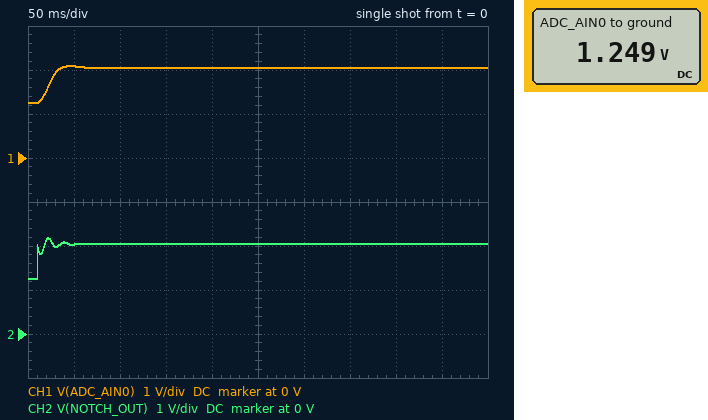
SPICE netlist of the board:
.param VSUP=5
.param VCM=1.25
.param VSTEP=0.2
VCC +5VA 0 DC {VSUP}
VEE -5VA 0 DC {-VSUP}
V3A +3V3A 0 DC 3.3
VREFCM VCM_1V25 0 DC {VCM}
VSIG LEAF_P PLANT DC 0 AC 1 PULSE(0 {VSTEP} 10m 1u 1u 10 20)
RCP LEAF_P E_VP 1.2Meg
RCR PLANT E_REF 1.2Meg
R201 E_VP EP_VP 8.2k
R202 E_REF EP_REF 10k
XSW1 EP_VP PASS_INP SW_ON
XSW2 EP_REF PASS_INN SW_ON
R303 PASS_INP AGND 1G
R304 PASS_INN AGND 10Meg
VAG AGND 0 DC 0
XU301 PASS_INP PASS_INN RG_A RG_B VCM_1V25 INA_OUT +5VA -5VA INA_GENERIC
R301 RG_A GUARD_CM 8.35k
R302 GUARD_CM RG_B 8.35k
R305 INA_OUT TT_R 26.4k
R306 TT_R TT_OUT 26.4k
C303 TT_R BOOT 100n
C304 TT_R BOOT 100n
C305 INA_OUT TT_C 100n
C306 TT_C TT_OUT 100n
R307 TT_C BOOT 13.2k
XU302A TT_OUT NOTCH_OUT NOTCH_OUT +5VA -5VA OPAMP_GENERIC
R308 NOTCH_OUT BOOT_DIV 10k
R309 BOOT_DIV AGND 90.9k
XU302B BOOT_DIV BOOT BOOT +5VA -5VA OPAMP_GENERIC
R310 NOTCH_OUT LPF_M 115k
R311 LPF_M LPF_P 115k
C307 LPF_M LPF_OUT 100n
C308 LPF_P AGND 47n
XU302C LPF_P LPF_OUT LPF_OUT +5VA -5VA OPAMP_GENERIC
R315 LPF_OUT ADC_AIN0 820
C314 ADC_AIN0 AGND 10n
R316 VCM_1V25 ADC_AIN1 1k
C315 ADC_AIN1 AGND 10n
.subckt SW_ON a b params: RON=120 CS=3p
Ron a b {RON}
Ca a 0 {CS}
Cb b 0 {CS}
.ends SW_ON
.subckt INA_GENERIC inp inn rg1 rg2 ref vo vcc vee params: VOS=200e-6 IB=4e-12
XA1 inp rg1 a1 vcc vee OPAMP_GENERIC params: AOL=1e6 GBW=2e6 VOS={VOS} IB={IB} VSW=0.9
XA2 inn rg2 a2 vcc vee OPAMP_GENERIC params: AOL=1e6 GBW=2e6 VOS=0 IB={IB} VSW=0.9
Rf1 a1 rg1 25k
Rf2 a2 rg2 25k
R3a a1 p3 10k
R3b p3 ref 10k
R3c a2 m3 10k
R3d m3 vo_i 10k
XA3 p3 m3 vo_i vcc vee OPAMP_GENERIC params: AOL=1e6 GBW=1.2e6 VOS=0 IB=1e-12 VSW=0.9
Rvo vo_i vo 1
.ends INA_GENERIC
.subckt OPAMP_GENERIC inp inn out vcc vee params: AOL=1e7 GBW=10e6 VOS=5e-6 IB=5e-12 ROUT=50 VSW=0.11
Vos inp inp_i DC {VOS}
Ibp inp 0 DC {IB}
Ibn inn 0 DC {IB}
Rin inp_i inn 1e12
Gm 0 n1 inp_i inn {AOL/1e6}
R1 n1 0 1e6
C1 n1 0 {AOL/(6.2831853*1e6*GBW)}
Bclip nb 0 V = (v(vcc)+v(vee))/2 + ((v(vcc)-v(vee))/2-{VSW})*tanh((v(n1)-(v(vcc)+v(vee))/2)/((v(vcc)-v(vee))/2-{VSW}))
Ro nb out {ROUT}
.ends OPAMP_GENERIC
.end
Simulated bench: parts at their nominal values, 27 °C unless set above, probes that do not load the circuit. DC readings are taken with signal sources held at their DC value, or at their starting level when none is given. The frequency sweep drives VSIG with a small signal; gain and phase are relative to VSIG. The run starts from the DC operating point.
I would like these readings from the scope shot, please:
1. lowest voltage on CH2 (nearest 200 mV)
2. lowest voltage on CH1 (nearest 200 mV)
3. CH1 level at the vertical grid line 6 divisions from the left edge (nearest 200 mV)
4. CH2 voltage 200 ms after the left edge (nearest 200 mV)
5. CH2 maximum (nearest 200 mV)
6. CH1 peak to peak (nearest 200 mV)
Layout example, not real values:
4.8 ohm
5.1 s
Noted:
1.2 V
1.2 V
2.0 V
2.0 V
2.2 V
800 mV
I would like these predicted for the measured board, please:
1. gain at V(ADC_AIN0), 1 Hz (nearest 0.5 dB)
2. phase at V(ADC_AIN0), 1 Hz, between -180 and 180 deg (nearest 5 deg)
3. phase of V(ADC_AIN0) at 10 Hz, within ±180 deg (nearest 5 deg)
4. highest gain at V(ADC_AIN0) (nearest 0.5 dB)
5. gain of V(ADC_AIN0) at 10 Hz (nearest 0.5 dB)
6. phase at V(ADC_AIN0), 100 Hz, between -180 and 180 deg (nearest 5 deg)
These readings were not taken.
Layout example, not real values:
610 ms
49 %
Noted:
12.0 dB
-5 deg
-45 deg
12.0 dB
12.0 dB
-145 deg
